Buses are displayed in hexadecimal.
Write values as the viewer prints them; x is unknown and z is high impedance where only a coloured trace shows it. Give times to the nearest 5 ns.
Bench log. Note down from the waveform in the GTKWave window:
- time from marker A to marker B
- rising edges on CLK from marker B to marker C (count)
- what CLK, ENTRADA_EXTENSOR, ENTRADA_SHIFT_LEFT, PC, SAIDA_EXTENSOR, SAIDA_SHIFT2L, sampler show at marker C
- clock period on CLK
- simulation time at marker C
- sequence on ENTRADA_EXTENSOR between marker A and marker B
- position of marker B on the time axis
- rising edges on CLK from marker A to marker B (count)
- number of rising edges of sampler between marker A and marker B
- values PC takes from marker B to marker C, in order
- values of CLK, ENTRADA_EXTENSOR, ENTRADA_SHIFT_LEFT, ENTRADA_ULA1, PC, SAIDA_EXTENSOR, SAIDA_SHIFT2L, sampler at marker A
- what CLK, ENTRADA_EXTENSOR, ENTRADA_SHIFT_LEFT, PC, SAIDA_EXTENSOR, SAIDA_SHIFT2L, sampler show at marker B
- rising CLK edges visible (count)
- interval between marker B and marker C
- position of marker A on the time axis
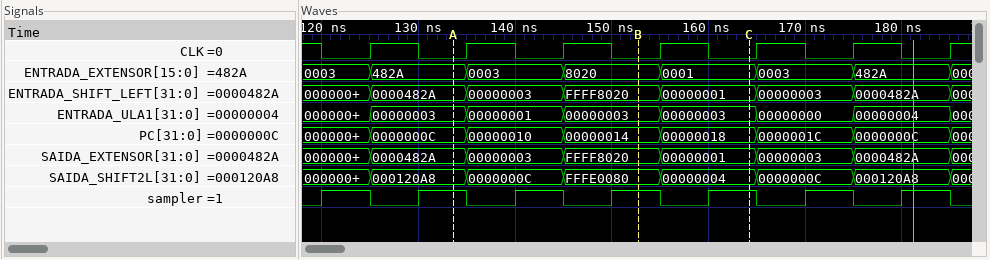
20 ns
1
CLK=0, ENTRADA_EXTENSOR=0001, ENTRADA_SHIFT_LEFT=00000001, PC=00000018, SAIDA_EXTENSOR=00000001, SAIDA_SHIFT2L=00000004, sampler=1
10 ns
165 ns
482A, 0003, 8020
155 ns
2
2
00000014, 00000018
CLK=0, ENTRADA_EXTENSOR=482A, ENTRADA_SHIFT_LEFT=0000482A, ENTRADA_ULA1=00000003, PC=0000000C, SAIDA_EXTENSOR=0000482A, SAIDA_SHIFT2L=000120A8, sampler=1
CLK=0, ENTRADA_EXTENSOR=8020, ENTRADA_SHIFT_LEFT=FFFF8020, PC=00000014, SAIDA_EXTENSOR=FFFF8020, SAIDA_SHIFT2L=FFFE0080, sampler=1
7
10 ns
135 ns
